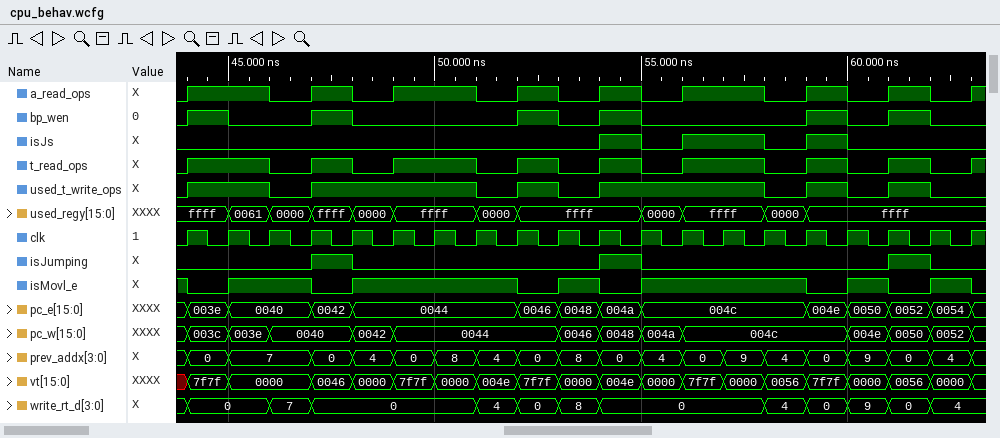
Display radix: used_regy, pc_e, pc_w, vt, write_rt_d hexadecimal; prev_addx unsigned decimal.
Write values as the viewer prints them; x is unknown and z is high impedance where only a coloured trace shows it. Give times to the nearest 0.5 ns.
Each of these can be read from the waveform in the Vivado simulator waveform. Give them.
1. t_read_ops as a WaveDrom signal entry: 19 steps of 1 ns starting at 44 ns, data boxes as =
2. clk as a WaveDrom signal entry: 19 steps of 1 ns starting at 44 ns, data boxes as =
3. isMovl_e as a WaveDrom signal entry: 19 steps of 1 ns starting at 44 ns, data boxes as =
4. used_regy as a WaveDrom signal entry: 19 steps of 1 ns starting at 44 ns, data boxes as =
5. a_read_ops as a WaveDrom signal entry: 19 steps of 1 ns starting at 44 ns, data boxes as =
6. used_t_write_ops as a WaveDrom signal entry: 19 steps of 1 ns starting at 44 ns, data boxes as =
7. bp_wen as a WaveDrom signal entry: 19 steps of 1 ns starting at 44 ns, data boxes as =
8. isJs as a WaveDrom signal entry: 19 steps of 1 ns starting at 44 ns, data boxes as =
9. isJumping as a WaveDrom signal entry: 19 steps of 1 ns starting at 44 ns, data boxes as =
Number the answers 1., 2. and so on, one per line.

1. {name: 't_read_ops', wave: '1.0101.010101.01010'}
2. {name: 'clk', wave: 'p..................'}
3. {name: 'isMovl_e', wave: '01.01...0101...0101'}
4. {name: 'used_regy', wave: '======.==..==.==...', data: 'ffff 0061 0000 ffff 0000 ffff 0000 ffff 0000 ffff 0000 ffff'}
5. {name: 'a_read_ops', wave: '1.0101.010101.01010'}
6. {name: 'used_t_write_ops', wave: '1.01...0101...01010'}
7. {name: 'bp_wen', wave: '10.10...1010...1010'}
8. {name: 'isJs', wave: '0.........101.010..'}
9. {name: 'isJumping', wave: '0..10.....10.....10'}
